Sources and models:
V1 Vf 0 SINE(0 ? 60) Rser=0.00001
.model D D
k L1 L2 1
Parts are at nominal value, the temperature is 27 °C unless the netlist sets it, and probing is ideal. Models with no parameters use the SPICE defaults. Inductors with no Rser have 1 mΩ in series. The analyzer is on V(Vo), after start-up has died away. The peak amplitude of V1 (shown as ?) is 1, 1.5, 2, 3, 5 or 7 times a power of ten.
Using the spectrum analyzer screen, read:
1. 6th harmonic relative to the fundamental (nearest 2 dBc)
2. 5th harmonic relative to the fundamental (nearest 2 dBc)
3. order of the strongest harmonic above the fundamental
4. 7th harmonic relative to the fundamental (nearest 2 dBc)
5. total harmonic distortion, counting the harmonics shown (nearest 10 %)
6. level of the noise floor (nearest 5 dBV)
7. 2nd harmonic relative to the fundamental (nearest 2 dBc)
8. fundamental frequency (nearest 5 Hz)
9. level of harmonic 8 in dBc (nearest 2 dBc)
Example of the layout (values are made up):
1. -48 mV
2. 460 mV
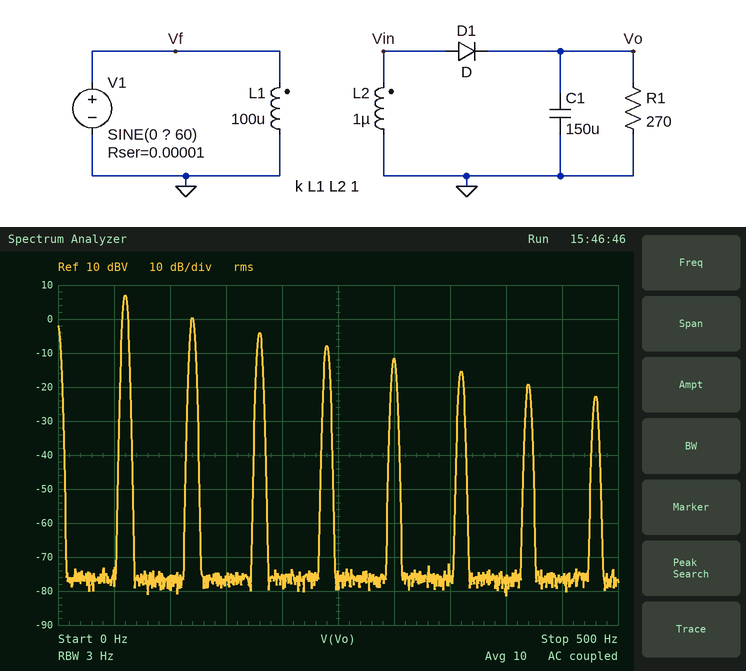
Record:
1. -22 dBc
2. -18 dBc
3. 2
4. -26 dBc
5. 60 %
6. -75 dBV
7. -6 dBc
8. 60 Hz
9. -30 dBc
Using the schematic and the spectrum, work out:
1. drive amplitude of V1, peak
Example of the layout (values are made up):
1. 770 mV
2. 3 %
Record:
1. 300 V
